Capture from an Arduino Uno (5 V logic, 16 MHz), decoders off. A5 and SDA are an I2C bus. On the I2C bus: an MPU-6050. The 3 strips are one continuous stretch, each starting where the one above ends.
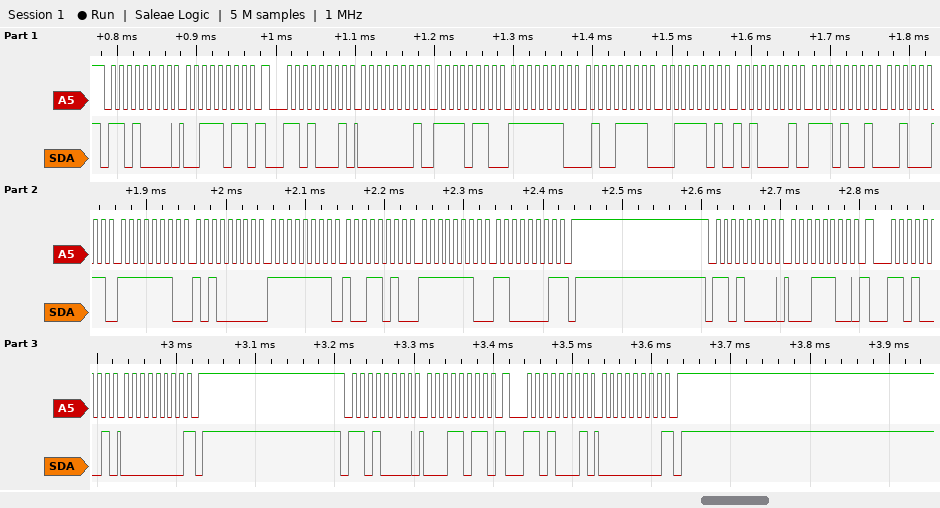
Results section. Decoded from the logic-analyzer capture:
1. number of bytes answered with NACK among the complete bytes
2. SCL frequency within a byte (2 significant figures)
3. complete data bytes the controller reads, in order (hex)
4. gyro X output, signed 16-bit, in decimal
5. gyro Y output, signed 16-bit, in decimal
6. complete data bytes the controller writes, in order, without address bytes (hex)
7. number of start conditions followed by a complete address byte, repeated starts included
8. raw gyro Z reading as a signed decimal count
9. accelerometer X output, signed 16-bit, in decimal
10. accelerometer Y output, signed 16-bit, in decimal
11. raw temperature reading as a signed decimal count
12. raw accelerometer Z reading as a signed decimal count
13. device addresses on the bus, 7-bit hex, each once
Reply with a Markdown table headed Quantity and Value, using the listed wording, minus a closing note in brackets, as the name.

| Quantity | Value |
|---|---|
| number of bytes answered with NACK among the complete bytes | 3 |
| SCL frequency within a byte | 100 kHz |
| complete data bytes the controller reads, in order | 01 F6 FE 4F 3D A1 E9 23 FE A0 FF 9A FE C1 00 00 |
| gyro X output, signed 16-bit, in decimal | -352 |
| gyro Y output, signed 16-bit, in decimal | -102 |
| complete data bytes the controller writes, in order, without address bytes | 3B 1C 1B |
| number of start conditions followed by a complete address byte, repeated starts included | 6 |
| raw gyro Z reading as a signed decimal count | -319 |
| accelerometer X output, signed 16-bit, in decimal | 502 |
| accelerometer Y output, signed 16-bit, in decimal | -433 |
| raw temperature reading as a signed decimal count | -5853 |
| raw accelerometer Z reading as a signed decimal count | 15777 |
| device addresses on the bus, 7-bit hex, each once | 0x68 |
